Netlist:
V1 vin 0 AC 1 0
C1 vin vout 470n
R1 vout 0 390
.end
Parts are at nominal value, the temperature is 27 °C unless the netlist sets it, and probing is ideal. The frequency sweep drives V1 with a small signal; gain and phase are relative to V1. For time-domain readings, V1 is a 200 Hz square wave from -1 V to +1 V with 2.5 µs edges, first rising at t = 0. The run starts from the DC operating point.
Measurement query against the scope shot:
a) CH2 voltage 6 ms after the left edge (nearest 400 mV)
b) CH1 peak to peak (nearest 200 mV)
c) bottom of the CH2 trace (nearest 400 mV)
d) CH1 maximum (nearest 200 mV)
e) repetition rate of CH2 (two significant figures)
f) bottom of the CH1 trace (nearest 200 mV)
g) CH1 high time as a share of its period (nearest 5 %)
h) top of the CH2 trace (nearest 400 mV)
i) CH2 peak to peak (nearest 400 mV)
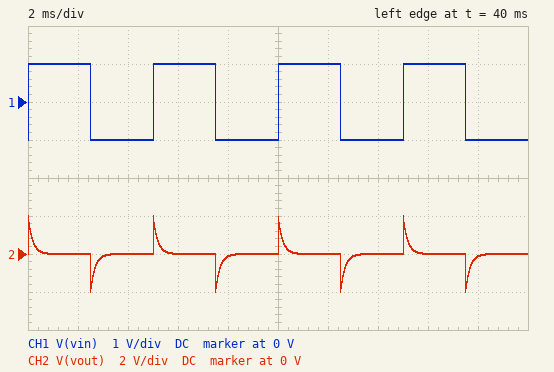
0 V
2.0 V
-2.0 V
1.0 V
200 Hz
-1.0 V
50 %
2.0 V
4.0 V
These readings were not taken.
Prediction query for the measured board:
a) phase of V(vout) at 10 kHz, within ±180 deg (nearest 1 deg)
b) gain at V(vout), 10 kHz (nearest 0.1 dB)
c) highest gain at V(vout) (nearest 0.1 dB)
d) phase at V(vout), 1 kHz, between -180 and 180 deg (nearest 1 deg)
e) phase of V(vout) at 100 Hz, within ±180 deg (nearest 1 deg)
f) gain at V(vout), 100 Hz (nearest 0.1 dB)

5 deg
0 dB
0 dB
41 deg
83 deg
-18.8 dB
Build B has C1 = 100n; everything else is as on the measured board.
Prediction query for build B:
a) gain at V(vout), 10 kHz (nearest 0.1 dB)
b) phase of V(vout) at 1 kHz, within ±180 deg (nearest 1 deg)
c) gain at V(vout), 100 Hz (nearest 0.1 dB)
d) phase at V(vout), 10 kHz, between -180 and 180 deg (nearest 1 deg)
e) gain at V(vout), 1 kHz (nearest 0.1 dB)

-0.7 dB
76 deg
-32.2 dB
22 deg
-12.5 dB
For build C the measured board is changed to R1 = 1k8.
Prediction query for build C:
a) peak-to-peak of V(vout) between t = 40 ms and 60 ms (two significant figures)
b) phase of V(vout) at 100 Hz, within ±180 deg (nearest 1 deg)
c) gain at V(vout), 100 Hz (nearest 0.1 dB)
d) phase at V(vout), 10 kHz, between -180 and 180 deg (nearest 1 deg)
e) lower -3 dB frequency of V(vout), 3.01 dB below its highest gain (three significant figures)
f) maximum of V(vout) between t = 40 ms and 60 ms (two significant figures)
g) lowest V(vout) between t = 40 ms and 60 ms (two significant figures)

3.8 V
62 deg
-6.6 dB
1 deg
188 Hz
1.9 V
-1.9 V
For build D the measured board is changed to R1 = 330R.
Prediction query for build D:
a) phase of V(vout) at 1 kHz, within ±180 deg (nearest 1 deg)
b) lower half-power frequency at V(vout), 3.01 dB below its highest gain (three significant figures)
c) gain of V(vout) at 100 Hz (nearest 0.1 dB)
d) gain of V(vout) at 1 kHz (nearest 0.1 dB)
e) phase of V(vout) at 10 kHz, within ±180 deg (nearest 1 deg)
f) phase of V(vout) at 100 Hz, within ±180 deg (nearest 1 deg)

46 deg
1.03 kHz
-20.3 dB
-3.1 dB
6 deg
84 deg
